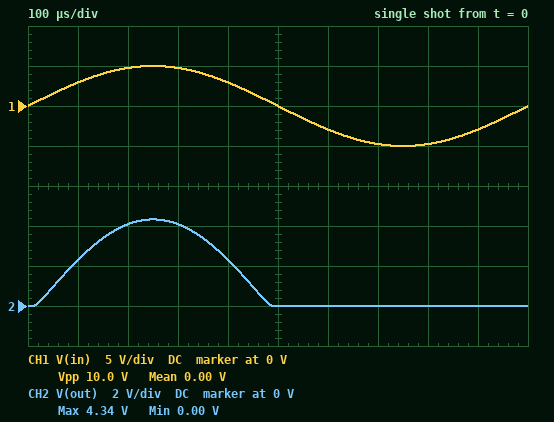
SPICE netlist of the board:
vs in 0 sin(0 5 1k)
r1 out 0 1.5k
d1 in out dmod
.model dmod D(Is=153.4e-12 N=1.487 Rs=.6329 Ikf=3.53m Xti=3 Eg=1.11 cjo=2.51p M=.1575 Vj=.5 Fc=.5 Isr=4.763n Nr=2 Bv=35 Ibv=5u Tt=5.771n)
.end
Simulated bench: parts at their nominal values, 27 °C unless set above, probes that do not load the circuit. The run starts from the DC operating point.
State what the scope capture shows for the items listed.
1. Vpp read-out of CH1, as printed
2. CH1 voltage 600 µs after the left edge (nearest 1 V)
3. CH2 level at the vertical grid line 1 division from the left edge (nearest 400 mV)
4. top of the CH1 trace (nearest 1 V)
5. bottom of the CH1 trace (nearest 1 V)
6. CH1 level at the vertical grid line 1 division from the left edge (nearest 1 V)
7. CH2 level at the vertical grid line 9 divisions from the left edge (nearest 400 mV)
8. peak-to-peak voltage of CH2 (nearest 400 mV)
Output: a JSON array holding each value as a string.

["10.0 V", "-3 V", "2.4 V", "5 V", "-5 V", "3 V", "0 V", "4.4 V"]
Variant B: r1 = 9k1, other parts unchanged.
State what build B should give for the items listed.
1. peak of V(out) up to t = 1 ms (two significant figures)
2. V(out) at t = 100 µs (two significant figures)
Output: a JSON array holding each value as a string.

["4.4 V", "2.4 V"]
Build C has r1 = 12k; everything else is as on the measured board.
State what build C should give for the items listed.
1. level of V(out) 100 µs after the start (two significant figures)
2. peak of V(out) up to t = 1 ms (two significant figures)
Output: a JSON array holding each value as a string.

["2.4 V", "4.4 V"]
